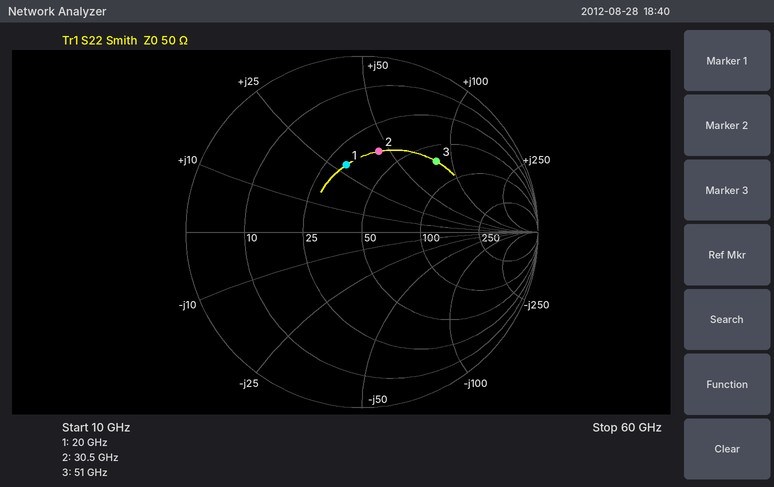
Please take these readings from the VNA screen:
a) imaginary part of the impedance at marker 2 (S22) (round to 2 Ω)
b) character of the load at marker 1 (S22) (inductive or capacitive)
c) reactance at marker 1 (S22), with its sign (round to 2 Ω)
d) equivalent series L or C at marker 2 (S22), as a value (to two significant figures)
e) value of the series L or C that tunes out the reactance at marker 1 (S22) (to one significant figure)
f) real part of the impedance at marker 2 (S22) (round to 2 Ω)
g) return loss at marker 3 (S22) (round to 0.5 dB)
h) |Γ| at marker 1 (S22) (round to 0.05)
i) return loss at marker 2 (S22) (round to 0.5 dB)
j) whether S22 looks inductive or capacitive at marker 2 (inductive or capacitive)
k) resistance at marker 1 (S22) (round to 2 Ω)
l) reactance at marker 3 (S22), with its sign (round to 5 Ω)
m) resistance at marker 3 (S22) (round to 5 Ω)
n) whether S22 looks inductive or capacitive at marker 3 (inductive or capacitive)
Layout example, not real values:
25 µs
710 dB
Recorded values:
+44 Ω
inductive
+28 Ω
230 pH
300 fF
38 Ω
4.5 dB
0.40
6.5 dB
inductive
32 Ω
+80 Ω
65 Ω
inductive
